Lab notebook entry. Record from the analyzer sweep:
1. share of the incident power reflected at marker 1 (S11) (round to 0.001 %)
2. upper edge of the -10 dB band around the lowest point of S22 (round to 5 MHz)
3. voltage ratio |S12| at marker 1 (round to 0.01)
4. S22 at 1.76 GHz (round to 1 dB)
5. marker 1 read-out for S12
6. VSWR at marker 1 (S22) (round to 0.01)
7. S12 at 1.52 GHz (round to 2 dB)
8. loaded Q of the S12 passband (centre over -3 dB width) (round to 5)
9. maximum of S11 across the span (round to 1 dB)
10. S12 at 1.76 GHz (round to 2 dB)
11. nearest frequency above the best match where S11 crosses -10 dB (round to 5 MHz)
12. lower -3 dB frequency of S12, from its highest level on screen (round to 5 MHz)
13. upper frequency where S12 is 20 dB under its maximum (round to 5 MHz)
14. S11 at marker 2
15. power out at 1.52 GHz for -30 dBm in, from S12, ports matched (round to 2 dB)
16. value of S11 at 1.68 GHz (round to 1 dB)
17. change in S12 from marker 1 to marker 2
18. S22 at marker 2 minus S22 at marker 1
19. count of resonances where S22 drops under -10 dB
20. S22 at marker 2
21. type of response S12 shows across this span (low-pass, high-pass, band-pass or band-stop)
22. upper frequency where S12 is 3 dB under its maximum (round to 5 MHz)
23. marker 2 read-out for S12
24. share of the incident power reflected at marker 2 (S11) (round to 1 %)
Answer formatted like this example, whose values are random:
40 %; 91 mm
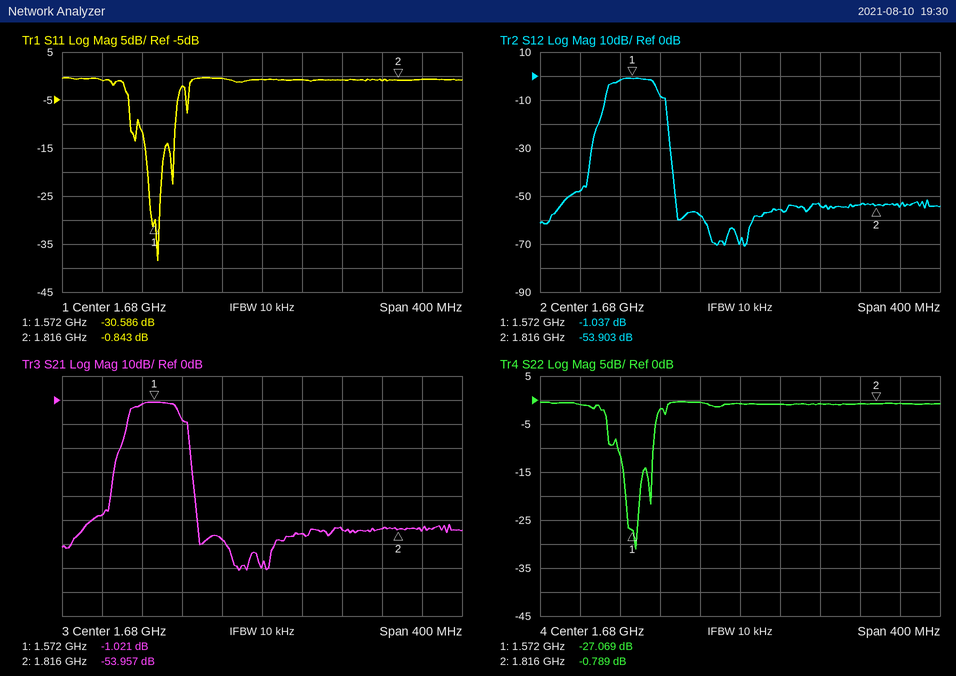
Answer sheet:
0.087 %; 1.595 GHz; 0.89; -1 dB; -1.037 dB; 1.09; -48 dB; 35; 0 dB; -54 dB; 1.595 GHz; 1.550 GHz; 1.610 GHz; -0.843 dB; -78 dBm; -1 dB; -52.866 dB; 26.280 dB; 2; -0.789 dB; band-pass; 1.595 GHz; -53.903 dB; 82 %
